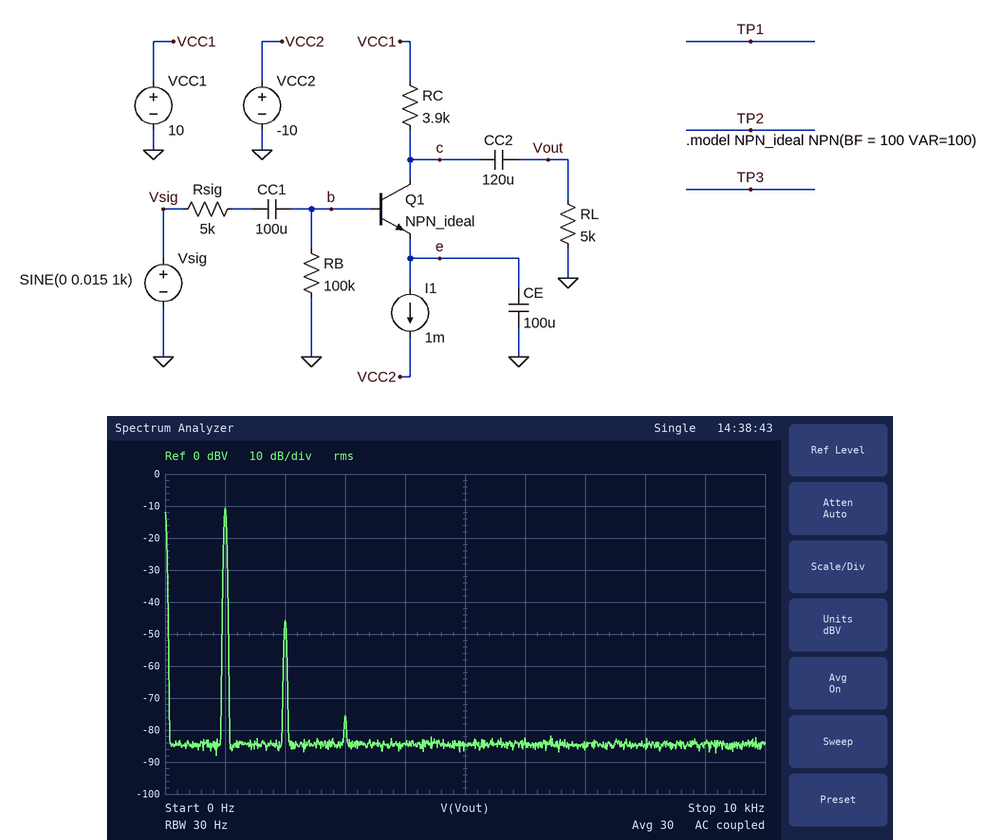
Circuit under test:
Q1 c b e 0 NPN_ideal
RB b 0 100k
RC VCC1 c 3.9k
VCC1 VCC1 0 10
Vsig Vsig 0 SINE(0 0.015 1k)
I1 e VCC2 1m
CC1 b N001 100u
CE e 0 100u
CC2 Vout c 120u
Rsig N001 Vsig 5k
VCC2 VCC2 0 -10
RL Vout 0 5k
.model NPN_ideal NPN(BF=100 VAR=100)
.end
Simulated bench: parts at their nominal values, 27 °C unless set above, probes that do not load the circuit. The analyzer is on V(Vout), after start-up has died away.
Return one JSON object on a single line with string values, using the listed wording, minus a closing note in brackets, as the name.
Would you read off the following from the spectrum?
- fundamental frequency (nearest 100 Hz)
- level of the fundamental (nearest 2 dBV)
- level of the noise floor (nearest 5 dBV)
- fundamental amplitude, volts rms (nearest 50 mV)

{"fundamental frequency": "1.0 kHz", "level of the fundamental": "-10 dBV", "level of the noise floor": "-85 dBV", "fundamental amplitude, volts rms": "300 mV"}
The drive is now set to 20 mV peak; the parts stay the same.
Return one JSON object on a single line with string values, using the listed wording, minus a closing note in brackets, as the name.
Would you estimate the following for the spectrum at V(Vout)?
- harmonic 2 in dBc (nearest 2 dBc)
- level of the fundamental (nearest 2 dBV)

{"harmonic 2 in dBc": "-32 dBc", "level of the fundamental": "-8 dBV"}
